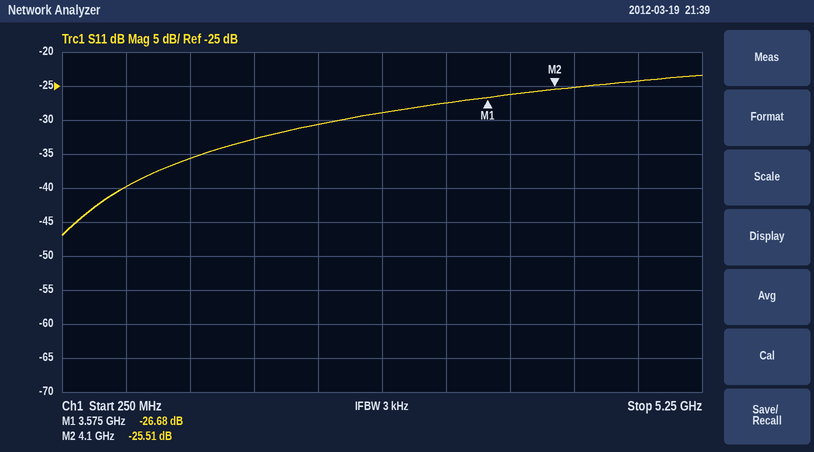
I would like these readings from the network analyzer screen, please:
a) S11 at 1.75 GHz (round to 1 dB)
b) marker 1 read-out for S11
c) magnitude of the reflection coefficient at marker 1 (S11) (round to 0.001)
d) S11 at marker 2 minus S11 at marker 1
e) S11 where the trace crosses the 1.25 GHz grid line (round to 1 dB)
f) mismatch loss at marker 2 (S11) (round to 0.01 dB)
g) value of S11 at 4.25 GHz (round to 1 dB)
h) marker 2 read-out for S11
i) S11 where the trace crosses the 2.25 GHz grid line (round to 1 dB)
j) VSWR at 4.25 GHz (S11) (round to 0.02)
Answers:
-33 dB
-26.68 dB
0.046
1.17 dB
-36 dB
0.01 dB
-25 dB
-25.51 dB
-31 dB
1.12
